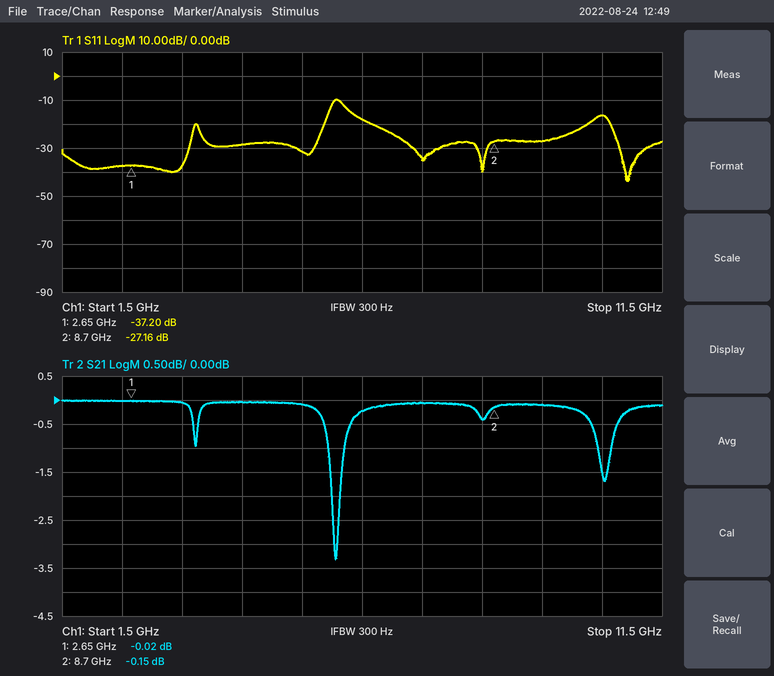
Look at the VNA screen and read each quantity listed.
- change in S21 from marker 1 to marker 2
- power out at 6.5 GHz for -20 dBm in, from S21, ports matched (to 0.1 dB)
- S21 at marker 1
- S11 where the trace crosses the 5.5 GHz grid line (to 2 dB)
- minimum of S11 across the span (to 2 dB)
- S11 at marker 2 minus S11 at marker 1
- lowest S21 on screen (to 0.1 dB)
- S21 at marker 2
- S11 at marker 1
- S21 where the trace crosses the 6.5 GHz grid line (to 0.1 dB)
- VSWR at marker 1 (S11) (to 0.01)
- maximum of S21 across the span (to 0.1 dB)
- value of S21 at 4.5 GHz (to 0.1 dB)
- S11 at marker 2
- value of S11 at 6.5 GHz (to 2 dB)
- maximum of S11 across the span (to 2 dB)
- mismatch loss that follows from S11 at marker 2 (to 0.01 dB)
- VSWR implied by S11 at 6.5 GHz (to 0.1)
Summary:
-0.13 dB
-20.2 dBm
-0.02 dB
-32 dB
-44 dB
10.04 dB
-3.3 dB
-0.15 dB
-37.20 dB
-0.2 dB
1.03
0.0 dB
0.0 dB
-27.16 dB
-18 dB
-10 dB
0.01 dB
1.3
